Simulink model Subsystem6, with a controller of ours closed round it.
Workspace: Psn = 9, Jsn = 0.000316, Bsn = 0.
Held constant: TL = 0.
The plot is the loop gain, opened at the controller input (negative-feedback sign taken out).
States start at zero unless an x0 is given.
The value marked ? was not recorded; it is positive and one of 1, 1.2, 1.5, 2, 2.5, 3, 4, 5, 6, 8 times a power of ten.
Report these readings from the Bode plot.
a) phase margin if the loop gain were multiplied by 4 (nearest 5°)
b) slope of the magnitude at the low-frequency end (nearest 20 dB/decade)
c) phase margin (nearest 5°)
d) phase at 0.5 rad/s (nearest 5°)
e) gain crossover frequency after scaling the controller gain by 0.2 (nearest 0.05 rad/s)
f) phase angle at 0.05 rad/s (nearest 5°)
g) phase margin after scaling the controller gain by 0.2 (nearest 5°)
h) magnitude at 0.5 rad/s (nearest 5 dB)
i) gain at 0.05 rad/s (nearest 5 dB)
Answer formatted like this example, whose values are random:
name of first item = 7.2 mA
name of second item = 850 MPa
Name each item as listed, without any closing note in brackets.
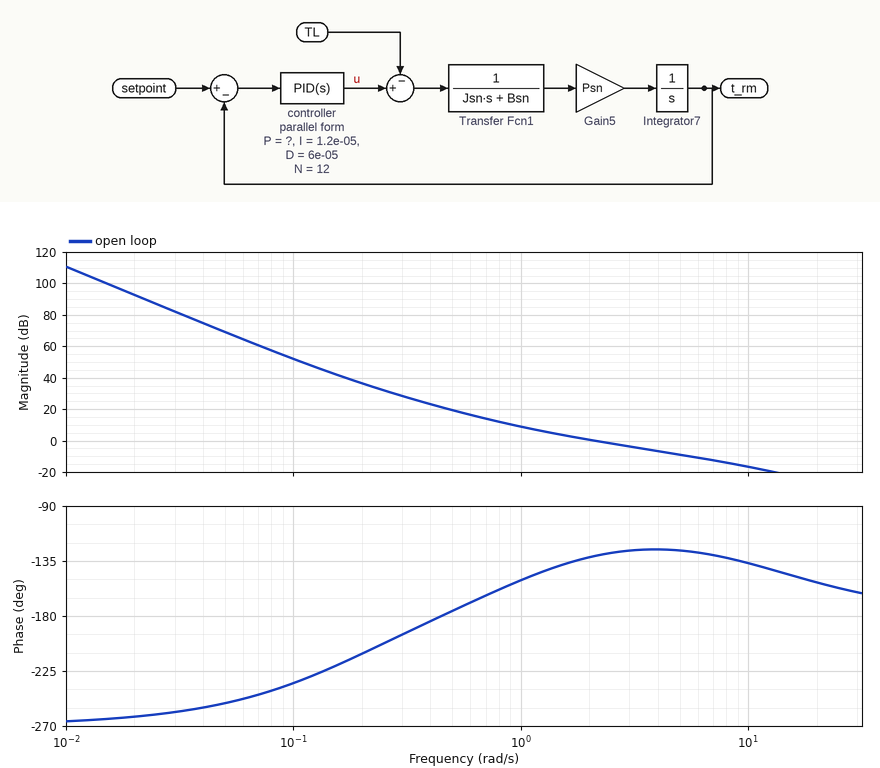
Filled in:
phase margin if the loop gain were multiplied by 4 = 50°
slope of the magnitude at the low-frequency end = -60 dB/decade
phase margin = 50°
phase at 0.5 rad/s = -175°
gain crossover frequency after scaling the controller gain by 0.2 = 0.70 rad/s
phase angle at 0.05 rad/s = -250°
phase margin after scaling the controller gain by 0.2 = 15°
magnitude at 0.5 rad/s = 20 dB
gain at 0.05 rad/s = 70 dB
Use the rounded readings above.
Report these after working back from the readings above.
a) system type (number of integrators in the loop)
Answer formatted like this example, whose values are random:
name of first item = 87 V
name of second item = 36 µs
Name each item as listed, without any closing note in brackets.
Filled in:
system type = 3
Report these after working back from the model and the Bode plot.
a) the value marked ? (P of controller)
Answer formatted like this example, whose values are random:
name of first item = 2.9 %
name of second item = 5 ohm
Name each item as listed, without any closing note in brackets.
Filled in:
the value marked ? = 8e-05
